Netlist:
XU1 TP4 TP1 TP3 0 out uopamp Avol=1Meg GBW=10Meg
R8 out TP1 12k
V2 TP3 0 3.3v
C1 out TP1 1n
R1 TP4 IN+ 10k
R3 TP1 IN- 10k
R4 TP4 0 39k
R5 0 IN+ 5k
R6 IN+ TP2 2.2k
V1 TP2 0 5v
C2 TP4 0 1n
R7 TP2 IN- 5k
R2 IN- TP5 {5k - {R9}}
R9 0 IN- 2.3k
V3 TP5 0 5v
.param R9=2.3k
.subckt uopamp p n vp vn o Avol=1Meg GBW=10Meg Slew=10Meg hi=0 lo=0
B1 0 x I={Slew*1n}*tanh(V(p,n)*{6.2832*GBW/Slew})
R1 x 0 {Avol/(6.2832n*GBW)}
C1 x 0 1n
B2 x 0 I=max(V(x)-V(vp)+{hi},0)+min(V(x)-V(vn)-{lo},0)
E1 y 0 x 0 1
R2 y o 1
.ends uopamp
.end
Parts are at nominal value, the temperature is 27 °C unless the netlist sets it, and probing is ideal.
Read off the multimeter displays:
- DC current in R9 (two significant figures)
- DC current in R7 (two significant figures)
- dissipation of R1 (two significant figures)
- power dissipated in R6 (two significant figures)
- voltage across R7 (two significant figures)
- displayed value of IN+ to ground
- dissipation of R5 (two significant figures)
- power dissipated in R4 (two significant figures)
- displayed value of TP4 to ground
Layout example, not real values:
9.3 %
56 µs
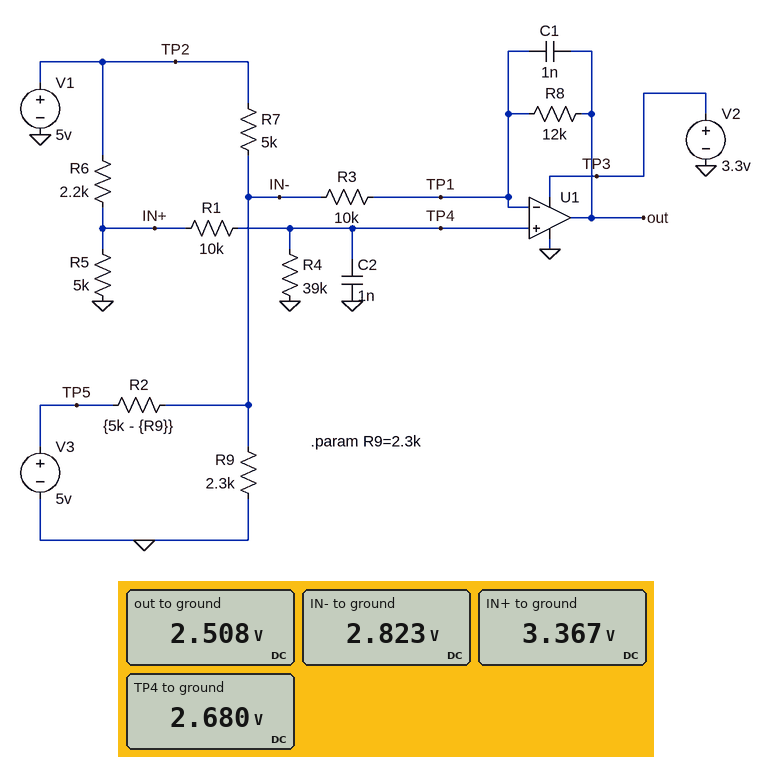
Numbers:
1.2 mA
440 µA
47 µW
1.2 mW
2.2 V
3.367 V
2.3 mW
180 µW
2.680 V
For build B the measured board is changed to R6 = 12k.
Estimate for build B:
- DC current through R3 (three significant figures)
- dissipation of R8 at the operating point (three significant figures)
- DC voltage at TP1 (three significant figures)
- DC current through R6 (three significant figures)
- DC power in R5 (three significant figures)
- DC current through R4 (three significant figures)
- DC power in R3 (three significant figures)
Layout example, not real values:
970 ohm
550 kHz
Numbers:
124 µA
184 µW
1.48 V
302 µA
376 µW
28.0 µA
153 µW
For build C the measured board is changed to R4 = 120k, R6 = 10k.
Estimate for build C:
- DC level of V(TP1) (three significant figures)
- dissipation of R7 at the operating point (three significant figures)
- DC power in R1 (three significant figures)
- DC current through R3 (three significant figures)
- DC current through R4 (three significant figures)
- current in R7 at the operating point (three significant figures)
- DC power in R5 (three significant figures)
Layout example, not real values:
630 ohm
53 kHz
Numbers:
1.50 V
1.04 mW
1.56 µW
122 µA
12.5 µA
457 µA
528 µW
